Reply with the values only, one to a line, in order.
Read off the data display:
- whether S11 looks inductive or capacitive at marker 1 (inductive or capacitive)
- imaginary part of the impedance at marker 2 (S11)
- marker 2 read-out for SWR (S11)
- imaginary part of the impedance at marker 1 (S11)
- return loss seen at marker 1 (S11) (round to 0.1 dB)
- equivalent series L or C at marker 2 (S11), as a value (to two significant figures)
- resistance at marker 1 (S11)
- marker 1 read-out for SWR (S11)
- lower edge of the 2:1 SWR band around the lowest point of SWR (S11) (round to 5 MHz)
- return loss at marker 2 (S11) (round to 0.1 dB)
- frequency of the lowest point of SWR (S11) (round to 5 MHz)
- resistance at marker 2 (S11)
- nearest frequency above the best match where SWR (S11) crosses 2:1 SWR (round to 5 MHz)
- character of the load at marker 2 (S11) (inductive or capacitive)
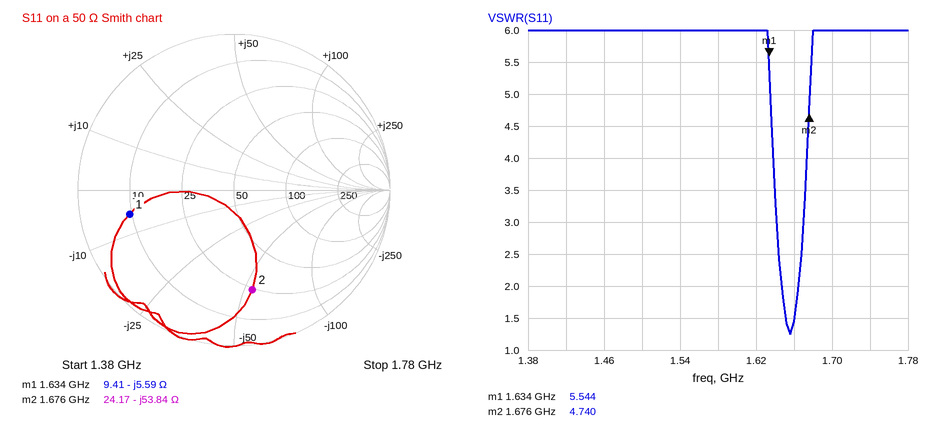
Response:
capacitive
-53.84 Ω
4.740
-5.59 Ω
3.3 dB
1.8 pF
9.41 Ω
5.544
1.645 GHz
3.7 dB
1.655 GHz
24.17 Ω
1.665 GHz
capacitive
